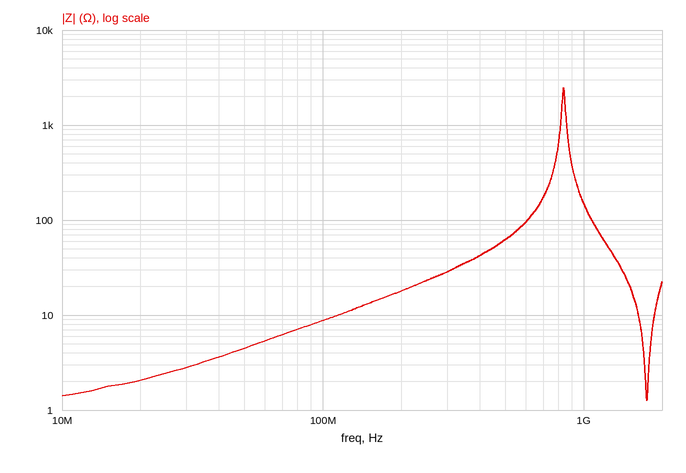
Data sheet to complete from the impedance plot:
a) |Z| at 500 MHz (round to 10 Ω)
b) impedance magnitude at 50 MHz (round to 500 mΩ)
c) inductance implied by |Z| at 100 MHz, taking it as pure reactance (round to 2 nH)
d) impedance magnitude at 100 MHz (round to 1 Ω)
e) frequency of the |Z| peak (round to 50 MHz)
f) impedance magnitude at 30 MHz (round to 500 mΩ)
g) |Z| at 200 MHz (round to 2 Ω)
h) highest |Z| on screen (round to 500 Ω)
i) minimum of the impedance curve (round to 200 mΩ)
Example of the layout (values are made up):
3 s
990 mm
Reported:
60 Ω
4.5 Ω
14 nH
9 Ω
850 MHz
3.0 Ω
18 Ω
2.5 kΩ
1.2 Ω
